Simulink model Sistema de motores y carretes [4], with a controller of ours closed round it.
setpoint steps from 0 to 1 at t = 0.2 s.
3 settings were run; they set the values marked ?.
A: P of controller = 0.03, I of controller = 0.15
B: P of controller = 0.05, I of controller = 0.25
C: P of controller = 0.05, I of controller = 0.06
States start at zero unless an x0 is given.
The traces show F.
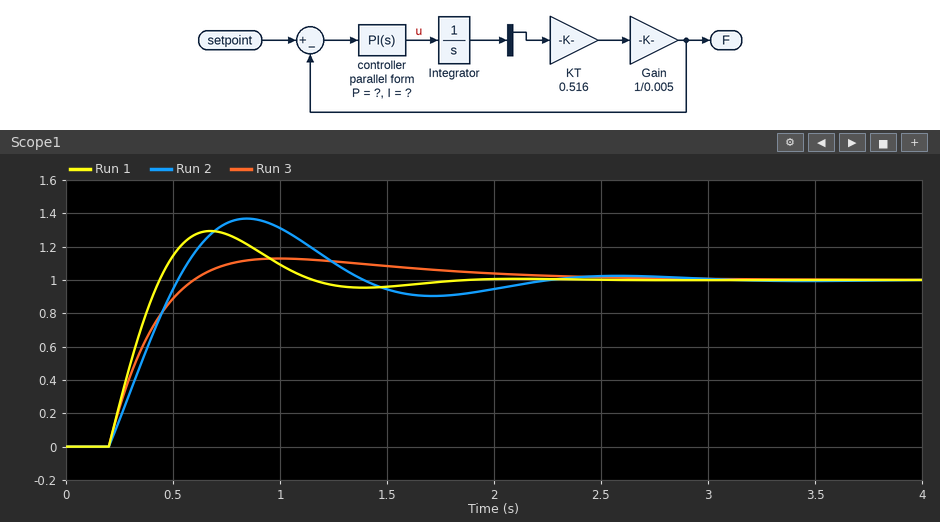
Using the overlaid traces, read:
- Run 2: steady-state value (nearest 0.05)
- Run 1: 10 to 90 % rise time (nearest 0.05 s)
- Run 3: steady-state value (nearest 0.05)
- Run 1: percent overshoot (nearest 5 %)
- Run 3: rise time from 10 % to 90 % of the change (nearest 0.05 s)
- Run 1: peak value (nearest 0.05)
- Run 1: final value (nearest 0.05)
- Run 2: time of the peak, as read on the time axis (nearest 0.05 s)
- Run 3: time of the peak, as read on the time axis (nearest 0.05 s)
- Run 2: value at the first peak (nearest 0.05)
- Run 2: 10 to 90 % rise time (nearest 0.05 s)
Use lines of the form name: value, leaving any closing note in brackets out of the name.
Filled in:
Run 2: steady-state value: 1.00
Run 1: 10 to 90 % rise time: 0.20 s
Run 3: steady-state value: 1.00
Run 1: percent overshoot: 30 %
Run 3: rise time from 10 % to 90 % of the change: 0.30 s
Run 1: peak value: 1.30
Run 1: final value: 1.00
Run 2: time of the peak, as read on the time axis: 0.85 s
Run 3: time of the peak, as read on the time axis: 1.00 s
Run 2: value at the first peak: 1.35
Run 2: 10 to 90 % rise time: 0.25 s
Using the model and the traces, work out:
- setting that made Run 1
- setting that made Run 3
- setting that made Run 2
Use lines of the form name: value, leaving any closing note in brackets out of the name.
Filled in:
setting that made Run 1: B
setting that made Run 3: C
setting that made Run 2: A
